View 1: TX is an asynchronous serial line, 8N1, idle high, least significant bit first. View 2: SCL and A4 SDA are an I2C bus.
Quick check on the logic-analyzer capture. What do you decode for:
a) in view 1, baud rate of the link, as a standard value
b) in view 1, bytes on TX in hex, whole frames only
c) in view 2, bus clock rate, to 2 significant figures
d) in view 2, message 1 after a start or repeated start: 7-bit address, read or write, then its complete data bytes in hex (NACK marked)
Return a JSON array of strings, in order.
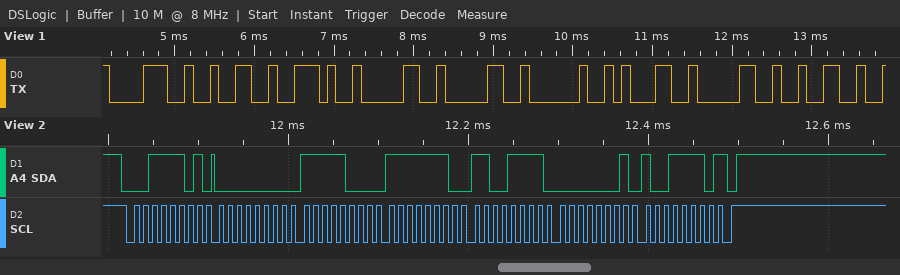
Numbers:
["9600 baud", "38 32 2E 30 30 20 31 30 32", "100 kHz", "0x1E read: 00 F8 FE CF 01 9E NACK"]
